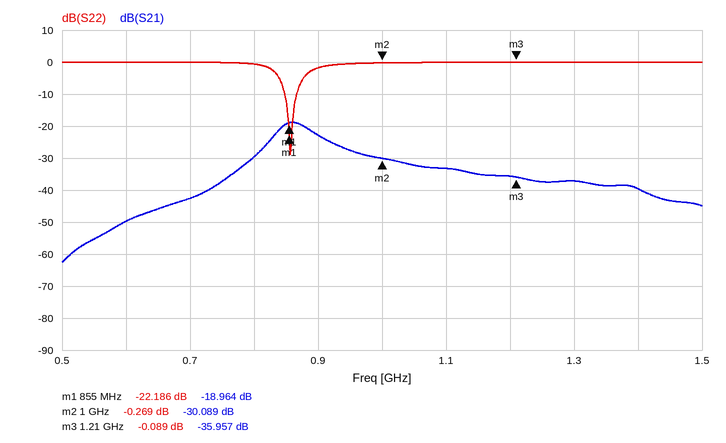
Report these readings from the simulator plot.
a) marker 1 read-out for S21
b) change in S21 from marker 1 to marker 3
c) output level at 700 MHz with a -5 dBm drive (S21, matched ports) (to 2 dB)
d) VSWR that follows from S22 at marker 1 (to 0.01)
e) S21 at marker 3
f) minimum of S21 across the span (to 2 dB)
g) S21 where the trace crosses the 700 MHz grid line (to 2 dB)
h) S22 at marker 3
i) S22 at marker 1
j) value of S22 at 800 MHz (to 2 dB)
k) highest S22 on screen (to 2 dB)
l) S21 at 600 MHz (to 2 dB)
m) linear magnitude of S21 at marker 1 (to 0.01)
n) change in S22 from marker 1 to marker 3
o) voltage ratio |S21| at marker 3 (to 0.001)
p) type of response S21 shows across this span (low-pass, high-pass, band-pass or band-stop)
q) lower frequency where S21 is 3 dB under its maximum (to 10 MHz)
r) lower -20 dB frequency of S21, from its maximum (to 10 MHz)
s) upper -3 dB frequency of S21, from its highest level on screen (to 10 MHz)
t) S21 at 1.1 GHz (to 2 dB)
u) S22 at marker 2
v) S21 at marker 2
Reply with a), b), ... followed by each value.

a) -18.964 dB
b) -16.993 dB
c) -48 dBm
d) 1.17
e) -35.957 dB
f) -62 dB
g) -42 dB
h) -0.089 dB
i) -22.186 dB
j) 0 dB
k) 0 dB
l) -50 dB
m) 0.11
n) 22.097 dB
o) 0.016
p) band-pass
q) 840 MHz
r) 740 MHz
s) 890 MHz
t) -34 dB
u) -0.269 dB
v) -30.089 dB
